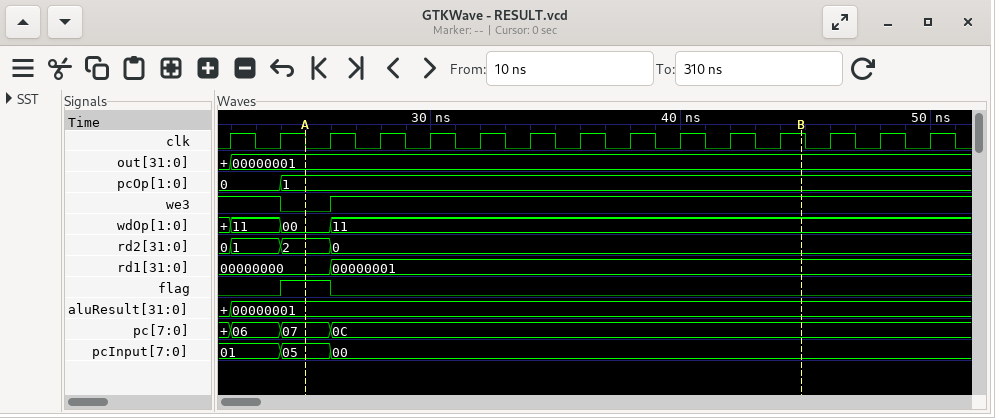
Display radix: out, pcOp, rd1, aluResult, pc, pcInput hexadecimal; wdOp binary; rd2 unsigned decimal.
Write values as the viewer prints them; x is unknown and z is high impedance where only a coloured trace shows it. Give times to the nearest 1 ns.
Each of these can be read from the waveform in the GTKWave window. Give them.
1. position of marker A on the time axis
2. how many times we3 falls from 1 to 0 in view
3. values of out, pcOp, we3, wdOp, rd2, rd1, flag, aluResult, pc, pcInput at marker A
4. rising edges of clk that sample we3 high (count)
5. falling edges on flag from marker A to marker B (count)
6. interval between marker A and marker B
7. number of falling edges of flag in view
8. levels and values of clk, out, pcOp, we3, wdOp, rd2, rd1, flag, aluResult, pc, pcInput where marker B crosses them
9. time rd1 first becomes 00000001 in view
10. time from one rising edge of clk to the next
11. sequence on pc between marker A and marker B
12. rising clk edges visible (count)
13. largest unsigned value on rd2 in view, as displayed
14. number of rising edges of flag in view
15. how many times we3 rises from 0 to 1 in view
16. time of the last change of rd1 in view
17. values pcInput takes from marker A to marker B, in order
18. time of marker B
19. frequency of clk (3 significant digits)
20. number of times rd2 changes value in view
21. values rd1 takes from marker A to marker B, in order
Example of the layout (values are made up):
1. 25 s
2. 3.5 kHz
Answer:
1. 25 ns
2. 1
3. out=00000001, pcOp=1, we3=0, wdOp=00, rd2=2, rd1=00000000, flag=1, aluResult=00000001, pc=07, pcInput=05
4. 14
5. 1
6. 20 ns
7. 1
8. clk=1, out=00000001, pcOp=1, we3=1, wdOp=11, rd2=0, rd1=00000001, flag=0, aluResult=00000001, pc=0C, pcInput=00
9. 26 ns
10. 2 ns
11. 07, 0C
12. 15
13. 2
14. 1
15. 1
16. 26 ns
17. 05, 00
18. 45 ns
19. 500 MHz
20. 3
21. 00000000, 00000001
